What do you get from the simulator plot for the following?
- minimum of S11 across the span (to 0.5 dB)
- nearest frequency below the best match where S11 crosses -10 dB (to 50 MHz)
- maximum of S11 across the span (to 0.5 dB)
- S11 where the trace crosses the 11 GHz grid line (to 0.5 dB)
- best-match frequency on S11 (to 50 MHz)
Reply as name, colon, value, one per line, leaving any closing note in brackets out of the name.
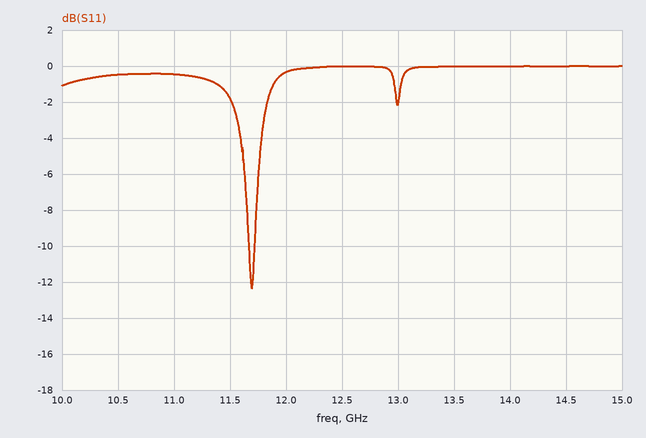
minimum of S11 across the span: -12.5 dB
nearest frequency below the best match where S11 crosses -10 dB: 11.65 GHz
maximum of S11 across the span: 0.0 dB
S11 where the trace crosses the 11 GHz grid line: -0.5 dB
best-match frequency on S11: 11.70 GHz
